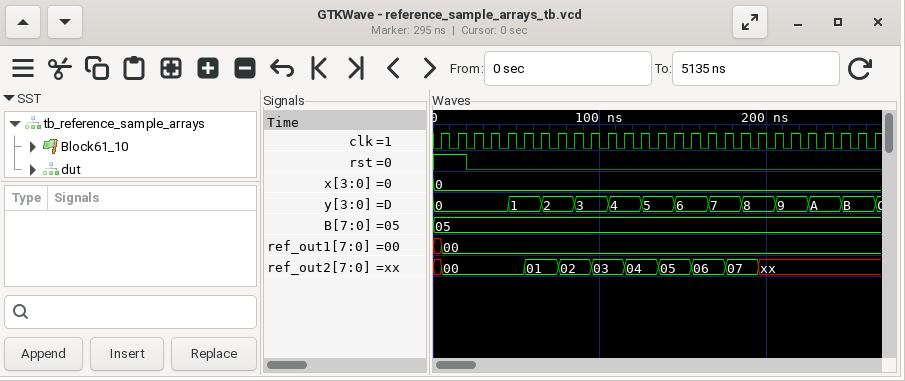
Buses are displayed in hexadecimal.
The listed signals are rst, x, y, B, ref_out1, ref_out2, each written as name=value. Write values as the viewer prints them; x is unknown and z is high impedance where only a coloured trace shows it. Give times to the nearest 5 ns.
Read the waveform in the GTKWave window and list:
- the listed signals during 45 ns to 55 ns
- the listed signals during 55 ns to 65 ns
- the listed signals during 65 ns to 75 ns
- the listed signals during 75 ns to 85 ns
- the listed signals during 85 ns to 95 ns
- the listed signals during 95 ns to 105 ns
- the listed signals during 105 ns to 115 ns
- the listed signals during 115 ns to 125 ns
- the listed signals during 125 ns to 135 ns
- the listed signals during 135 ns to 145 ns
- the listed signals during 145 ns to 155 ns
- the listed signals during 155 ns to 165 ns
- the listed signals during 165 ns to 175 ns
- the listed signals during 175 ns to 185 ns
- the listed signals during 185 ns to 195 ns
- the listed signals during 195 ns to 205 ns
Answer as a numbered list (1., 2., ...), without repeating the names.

1. rst=0, x=0, y=1, B=05, ref_out1=00, ref_out2=00
2. rst=0, x=0, y=1, B=05, ref_out1=00, ref_out2=01
3. rst=0, x=0, y=2, B=05, ref_out1=00, ref_out2=01
4. rst=0, x=0, y=2, B=05, ref_out1=00, ref_out2=02
5. rst=0, x=0, y=3, B=05, ref_out1=00, ref_out2=02
6. rst=0, x=0, y=3, B=05, ref_out1=00, ref_out2=03
7. rst=0, x=0, y=4, B=05, ref_out1=00, ref_out2=03
8. rst=0, x=0, y=4, B=05, ref_out1=00, ref_out2=04
9. rst=0, x=0, y=5, B=05, ref_out1=00, ref_out2=04
10. rst=0, x=0, y=5, B=05, ref_out1=00, ref_out2=05
11. rst=0, x=0, y=6, B=05, ref_out1=00, ref_out2=05
12. rst=0, x=0, y=6, B=05, ref_out1=00, ref_out2=06
13. rst=0, x=0, y=7, B=05, ref_out1=00, ref_out2=06
14. rst=0, x=0, y=7, B=05, ref_out1=00, ref_out2=07
15. rst=0, x=0, y=8, B=05, ref_out1=00, ref_out2=07
16. rst=0, x=0, y=8, B=05, ref_out1=00, ref_out2=xx
